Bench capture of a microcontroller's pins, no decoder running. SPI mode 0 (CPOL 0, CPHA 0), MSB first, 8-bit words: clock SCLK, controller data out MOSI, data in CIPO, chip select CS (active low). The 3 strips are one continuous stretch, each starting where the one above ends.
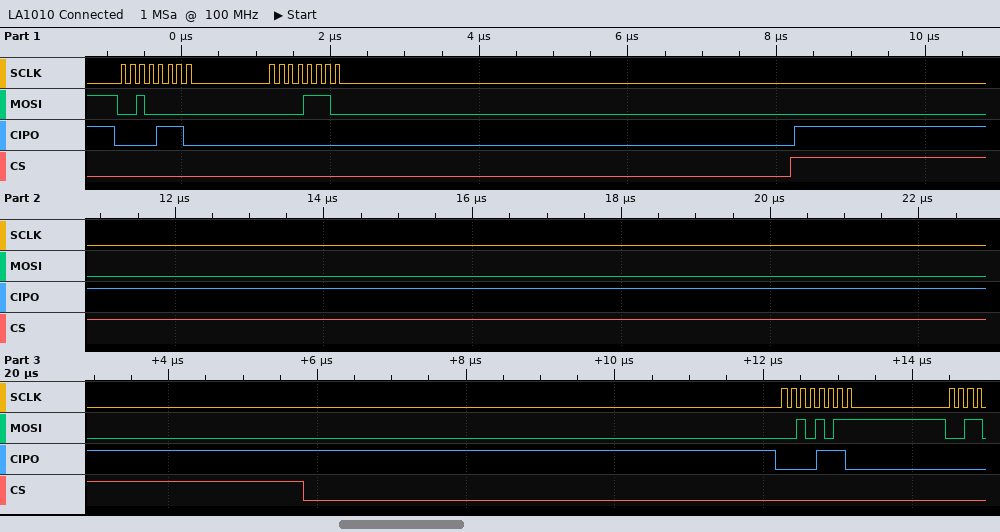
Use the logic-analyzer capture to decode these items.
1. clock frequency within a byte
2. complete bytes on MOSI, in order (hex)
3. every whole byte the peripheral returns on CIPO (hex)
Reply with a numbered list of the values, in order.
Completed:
1. 8 MHz
2. 0x20 0x0E 0x2B
3. 0x0E 0x00 0x0E
